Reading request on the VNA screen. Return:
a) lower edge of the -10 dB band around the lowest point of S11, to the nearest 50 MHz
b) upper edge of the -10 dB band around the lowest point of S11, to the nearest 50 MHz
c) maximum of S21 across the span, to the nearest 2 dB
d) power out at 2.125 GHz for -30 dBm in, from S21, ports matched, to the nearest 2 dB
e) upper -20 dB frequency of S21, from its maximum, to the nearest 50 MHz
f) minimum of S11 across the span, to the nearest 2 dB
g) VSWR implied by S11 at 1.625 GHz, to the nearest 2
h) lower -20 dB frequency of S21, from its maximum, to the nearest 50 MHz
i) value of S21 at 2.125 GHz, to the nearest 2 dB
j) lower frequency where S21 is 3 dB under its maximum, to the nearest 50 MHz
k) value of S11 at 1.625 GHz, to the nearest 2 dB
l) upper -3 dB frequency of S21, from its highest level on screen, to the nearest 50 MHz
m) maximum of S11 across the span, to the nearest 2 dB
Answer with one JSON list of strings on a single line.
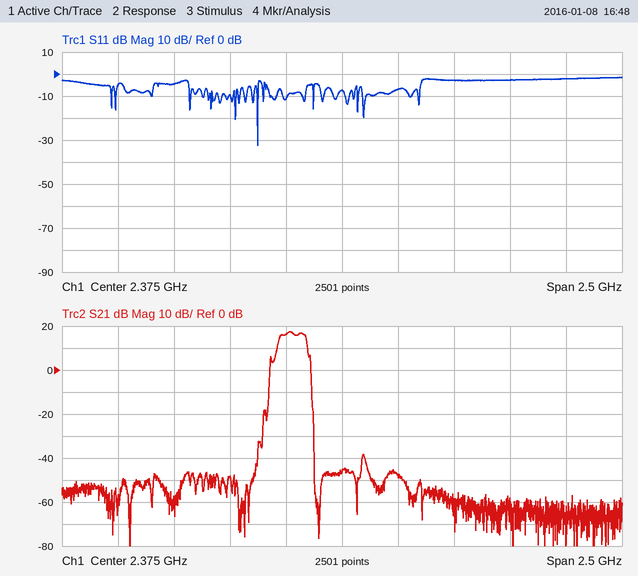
["2.00 GHz", "2.00 GHz", "18 dB", "-14 dBm", "2.25 GHz", "-32 dB", "4", "2.05 GHz", "16 dB", "2.10 GHz", "-4 dB", "2.20 GHz", "-2 dB"]
